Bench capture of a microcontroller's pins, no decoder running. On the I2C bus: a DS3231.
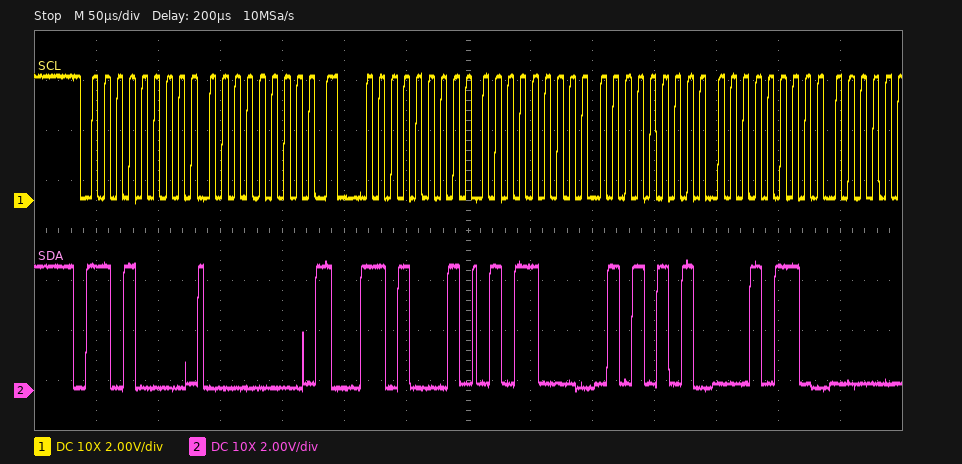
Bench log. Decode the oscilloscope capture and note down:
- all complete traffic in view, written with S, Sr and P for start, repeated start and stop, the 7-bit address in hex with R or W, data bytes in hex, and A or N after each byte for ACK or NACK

S 68W A 00 A Sr 68R A 58 A 55 A 16 A
